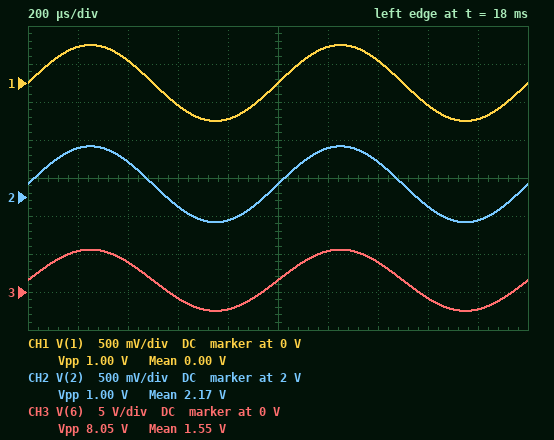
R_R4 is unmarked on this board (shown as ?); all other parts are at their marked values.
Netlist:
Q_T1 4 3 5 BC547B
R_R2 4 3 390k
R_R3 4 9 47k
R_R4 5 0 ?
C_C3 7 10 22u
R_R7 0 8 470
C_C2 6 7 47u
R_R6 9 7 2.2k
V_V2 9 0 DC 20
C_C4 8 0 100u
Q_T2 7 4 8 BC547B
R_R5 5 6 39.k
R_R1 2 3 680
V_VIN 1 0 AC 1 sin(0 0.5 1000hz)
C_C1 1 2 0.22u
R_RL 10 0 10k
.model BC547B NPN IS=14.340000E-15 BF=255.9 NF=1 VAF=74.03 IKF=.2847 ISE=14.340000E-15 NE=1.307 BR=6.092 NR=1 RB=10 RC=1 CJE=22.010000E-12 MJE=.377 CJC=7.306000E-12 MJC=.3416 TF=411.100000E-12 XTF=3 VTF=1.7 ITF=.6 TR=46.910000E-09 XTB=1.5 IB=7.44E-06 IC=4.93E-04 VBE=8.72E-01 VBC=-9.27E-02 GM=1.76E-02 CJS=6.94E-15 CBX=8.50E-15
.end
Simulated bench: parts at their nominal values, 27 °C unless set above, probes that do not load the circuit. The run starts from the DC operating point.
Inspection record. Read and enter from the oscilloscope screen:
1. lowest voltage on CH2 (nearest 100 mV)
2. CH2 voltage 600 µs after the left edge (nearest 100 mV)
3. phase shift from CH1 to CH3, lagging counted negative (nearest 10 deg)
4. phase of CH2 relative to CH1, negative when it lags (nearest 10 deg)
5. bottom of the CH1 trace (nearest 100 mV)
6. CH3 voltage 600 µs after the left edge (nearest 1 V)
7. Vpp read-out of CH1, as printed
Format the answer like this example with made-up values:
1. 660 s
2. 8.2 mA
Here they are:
1. 1.7 V
2. 1.9 V
3. 0 deg
4. 0 deg
5. -500 mV
6. -1 V
7. 1.00 V
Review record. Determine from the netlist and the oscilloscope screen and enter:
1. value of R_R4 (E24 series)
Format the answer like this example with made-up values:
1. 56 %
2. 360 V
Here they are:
1. 4.7 kΩ
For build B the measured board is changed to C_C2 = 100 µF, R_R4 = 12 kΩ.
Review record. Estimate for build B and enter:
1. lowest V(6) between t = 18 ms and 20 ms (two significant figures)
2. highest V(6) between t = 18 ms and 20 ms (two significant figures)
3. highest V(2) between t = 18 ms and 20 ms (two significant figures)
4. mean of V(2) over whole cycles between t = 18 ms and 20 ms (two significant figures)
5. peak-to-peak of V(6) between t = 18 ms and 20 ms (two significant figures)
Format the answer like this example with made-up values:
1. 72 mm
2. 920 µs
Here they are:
1. 2.9 V
2. 3.0 V
3. 4.0 V
4. 3.5 V
5. 120 mV
